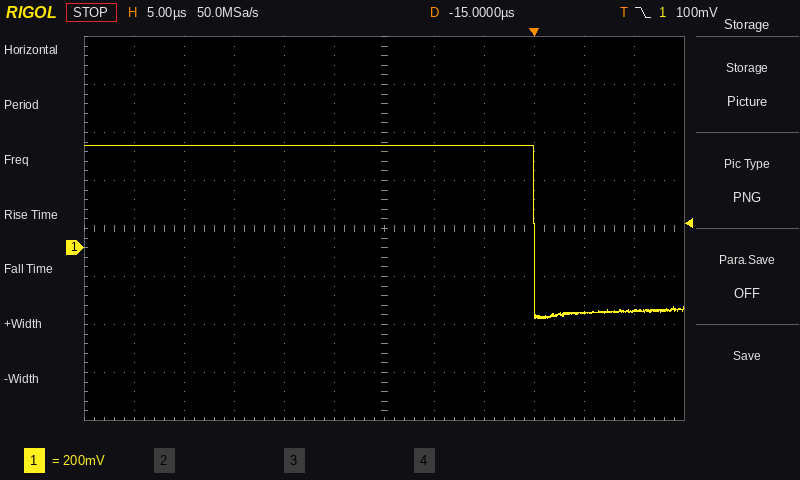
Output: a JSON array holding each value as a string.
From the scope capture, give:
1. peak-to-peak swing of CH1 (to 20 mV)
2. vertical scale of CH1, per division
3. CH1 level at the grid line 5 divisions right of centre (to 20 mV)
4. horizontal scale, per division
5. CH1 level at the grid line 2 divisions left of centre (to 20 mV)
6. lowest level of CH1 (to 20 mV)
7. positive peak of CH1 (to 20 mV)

["720 mV", "200 mV", "-260 mV", "5 µs", "420 mV", "-300 mV", "420 mV"]
